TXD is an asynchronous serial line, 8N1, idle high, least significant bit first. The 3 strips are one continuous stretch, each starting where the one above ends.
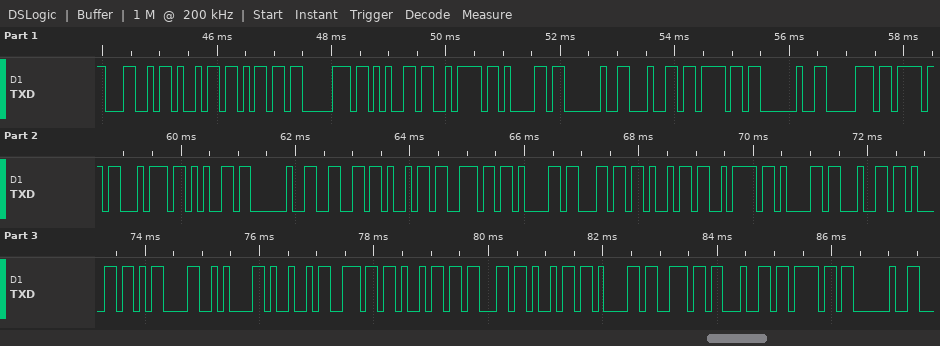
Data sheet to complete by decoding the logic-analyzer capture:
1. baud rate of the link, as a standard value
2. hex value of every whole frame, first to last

9600 baud
4C 69 6D 70 65 7A 61 20 64 6F 20 70 6F 74 65 20 66 69 6E 61 6C 69 7A 61 64 61 0D 0A 49 6E 69 63 69 61 6E 64 6F 20
